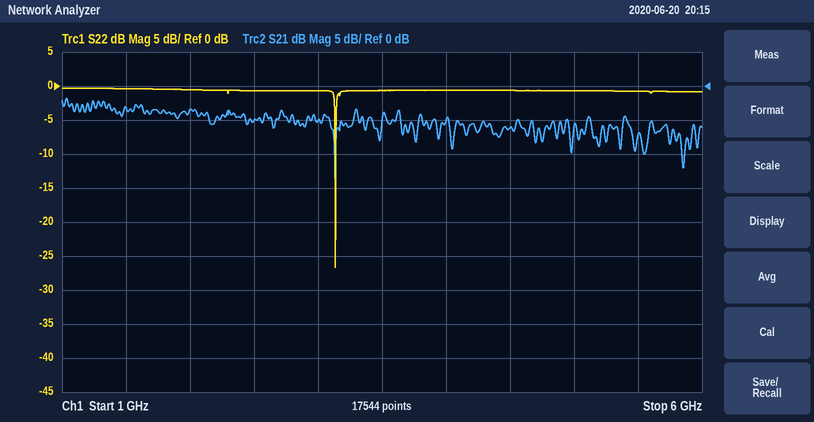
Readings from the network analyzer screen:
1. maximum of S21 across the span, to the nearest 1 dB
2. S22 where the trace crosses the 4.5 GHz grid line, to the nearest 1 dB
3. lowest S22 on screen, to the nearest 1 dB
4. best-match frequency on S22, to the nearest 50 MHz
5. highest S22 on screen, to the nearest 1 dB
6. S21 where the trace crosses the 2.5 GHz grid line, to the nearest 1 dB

-2 dB
-1 dB
-27 dB
3.15 GHz
0 dB
-5 dB
